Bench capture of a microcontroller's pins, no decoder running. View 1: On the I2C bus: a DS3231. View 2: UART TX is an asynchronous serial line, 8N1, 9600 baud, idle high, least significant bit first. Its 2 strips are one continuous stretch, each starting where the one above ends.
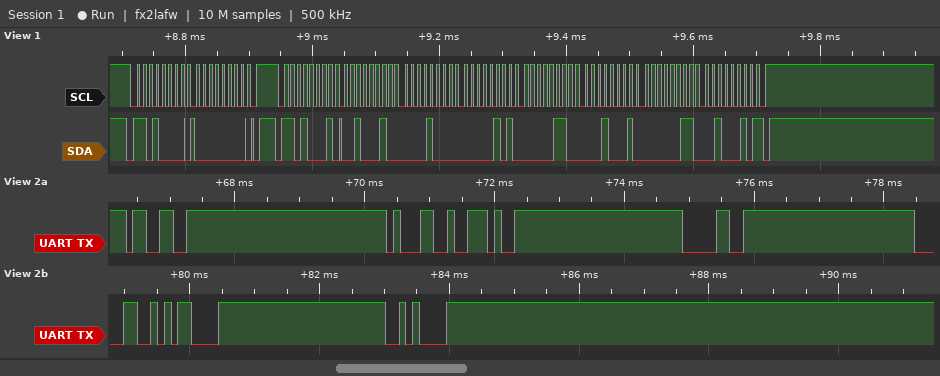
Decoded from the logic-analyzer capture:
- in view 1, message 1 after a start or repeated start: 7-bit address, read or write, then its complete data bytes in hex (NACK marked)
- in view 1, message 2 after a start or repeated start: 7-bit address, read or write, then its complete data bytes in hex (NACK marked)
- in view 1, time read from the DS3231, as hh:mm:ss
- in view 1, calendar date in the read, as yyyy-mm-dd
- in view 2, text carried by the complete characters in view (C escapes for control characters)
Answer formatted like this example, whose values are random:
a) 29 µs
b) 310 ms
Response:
a) 0x68 write: 00
b) 0x68 read: 22 08 05 06 11 03 22 NACK
c) 05:08:22
d) 2022-03-11
e) "31.00\r\n"
